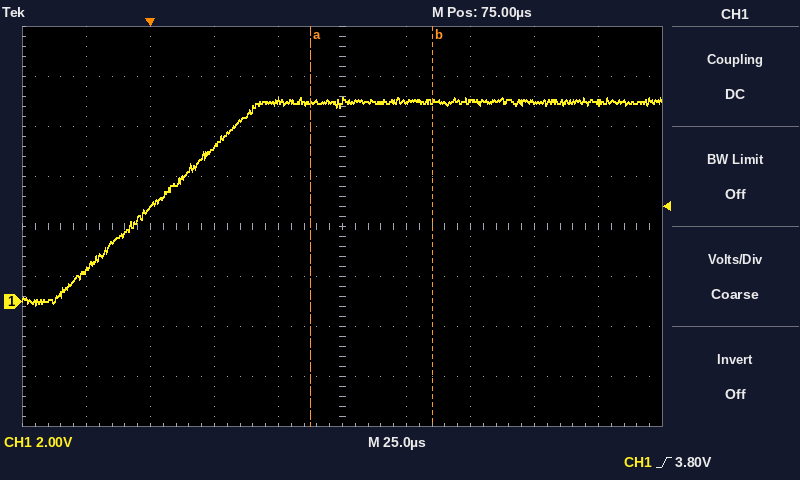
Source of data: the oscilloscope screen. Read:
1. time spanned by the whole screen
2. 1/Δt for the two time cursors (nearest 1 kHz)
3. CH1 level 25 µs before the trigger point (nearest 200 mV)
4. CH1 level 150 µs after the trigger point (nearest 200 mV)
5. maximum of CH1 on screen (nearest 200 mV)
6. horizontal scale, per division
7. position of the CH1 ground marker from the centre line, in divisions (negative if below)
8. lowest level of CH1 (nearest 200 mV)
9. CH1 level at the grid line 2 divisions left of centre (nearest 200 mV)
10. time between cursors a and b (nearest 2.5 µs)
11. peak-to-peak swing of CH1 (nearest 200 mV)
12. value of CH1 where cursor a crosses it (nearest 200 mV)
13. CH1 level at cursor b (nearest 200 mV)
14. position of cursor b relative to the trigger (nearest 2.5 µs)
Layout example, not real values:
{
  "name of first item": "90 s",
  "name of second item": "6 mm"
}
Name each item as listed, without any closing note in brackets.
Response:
{
  "time spanned by the whole screen": "250 µs",
  "1/Δt for the two time cursors": "21 kHz",
  "CH1 level 25 µs before the trigger point": "1.2 V",
  "CH1 level 150 µs after the trigger point": "8.0 V",
  "maximum of CH1 on screen": "8.2 V",
  "horizontal scale, per division": "25 µs",
  "position of the CH1 ground marker from the centre line, in divisions": "-1.5 div",
  "lowest level of CH1": "-200 mV",
  "CH1 level at the grid line 2 divisions left of centre": "6.2 V",
  "time between cursors a and b": "47.5 µs",
  "peak-to-peak swing of CH1": "8.4 V",
  "value of CH1 where cursor a crosses it": "8.0 V",
  "CH1 level at cursor b": "8.0 V",
  "position of cursor b relative to the trigger": "+110.0 µs"
}
